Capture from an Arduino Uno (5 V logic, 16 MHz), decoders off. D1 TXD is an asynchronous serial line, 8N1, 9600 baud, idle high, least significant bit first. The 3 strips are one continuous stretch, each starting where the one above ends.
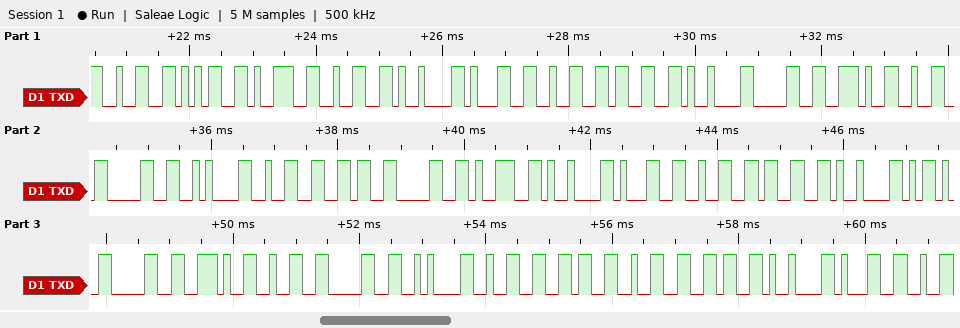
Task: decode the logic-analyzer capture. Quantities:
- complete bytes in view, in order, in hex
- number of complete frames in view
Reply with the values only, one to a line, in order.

32 35 39 32 09 31 32 33 09 30 2E 32 30 0A 32 36 30 39 09 31 32 33 09 2D 30 2E 32 30 0A 32 36 32 36 09 31
35
